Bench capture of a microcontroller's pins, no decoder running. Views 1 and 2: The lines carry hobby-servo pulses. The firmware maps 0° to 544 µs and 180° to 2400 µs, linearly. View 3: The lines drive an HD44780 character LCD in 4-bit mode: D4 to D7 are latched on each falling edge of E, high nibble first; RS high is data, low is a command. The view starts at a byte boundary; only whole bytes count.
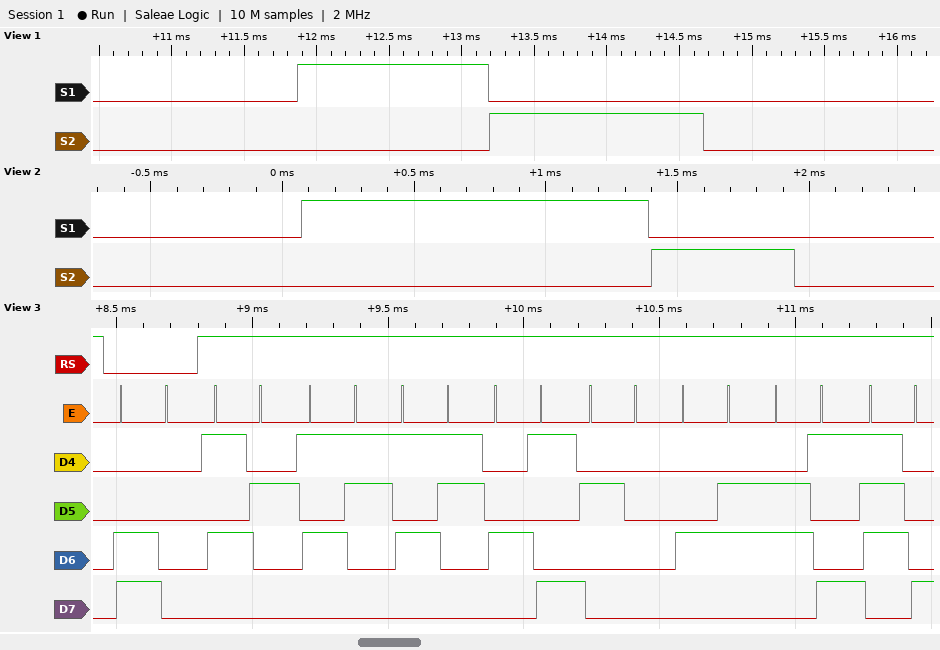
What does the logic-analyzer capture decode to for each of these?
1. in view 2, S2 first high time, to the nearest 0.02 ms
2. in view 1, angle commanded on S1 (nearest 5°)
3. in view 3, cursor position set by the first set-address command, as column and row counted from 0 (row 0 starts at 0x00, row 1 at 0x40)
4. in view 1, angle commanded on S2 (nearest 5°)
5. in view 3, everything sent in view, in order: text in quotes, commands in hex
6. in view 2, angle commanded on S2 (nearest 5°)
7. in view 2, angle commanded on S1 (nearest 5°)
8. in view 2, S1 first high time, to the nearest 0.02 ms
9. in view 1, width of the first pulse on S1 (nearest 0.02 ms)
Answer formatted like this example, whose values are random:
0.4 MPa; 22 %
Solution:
0.54 ms; 75°; column 0, row 1; 90°; 0xC0 "RSSI Fix"; 0°; 75°; 1.32 ms; 1.32 ms
